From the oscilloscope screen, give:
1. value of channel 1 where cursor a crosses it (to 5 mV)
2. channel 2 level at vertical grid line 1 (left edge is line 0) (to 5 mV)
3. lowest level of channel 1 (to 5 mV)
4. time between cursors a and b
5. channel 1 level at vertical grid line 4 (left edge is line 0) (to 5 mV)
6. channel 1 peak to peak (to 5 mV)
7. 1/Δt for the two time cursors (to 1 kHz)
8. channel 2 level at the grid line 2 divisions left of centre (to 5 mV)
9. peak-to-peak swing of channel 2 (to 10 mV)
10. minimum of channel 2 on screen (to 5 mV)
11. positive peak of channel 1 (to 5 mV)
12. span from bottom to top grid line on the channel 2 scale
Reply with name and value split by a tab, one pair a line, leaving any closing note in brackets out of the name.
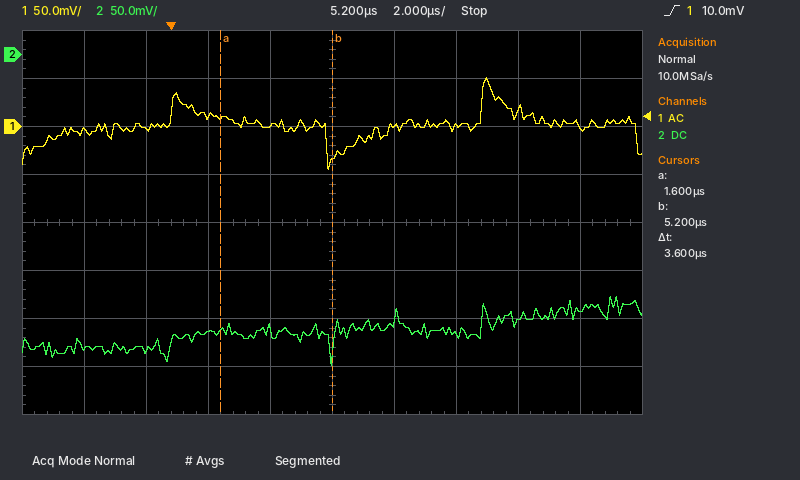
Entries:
value of channel 1 where cursor a crosses it	10 mV
channel 2 level at vertical grid line 1 (left edge is line 0)	-305 mV
lowest level of channel 1	-45 mV
time between cursors a and b	3.6 µs
channel 1 level at vertical grid line 4 (left edge is line 0)	0 mV
channel 1 peak to peak	95 mV
1/Δt for the two time cursors	278 kHz
channel 2 level at the grid line 2 divisions left of centre	-290 mV
peak-to-peak swing of channel 2	70 mV
minimum of channel 2 on screen	-325 mV
positive peak of channel 1	50 mV
span from bottom to top grid line on the channel 2 scale	400 mV
